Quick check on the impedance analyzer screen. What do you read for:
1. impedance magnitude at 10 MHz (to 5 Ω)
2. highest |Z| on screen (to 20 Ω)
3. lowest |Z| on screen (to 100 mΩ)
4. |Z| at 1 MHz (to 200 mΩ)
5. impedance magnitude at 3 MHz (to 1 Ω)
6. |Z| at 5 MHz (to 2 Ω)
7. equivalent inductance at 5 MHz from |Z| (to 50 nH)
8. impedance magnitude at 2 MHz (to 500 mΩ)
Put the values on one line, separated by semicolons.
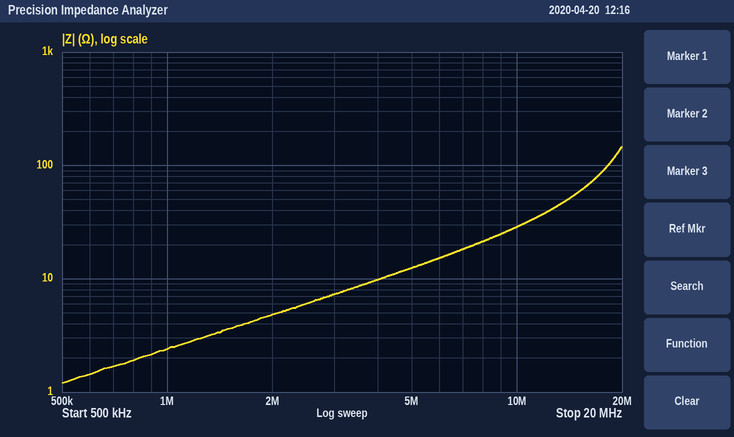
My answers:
30 Ω; 140 Ω; 1.2 Ω; 2.4 Ω; 7 Ω; 12 Ω; 400 nH; 5.0 Ω
